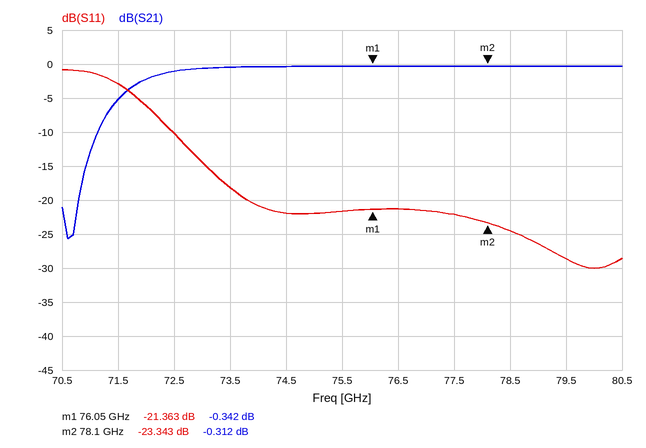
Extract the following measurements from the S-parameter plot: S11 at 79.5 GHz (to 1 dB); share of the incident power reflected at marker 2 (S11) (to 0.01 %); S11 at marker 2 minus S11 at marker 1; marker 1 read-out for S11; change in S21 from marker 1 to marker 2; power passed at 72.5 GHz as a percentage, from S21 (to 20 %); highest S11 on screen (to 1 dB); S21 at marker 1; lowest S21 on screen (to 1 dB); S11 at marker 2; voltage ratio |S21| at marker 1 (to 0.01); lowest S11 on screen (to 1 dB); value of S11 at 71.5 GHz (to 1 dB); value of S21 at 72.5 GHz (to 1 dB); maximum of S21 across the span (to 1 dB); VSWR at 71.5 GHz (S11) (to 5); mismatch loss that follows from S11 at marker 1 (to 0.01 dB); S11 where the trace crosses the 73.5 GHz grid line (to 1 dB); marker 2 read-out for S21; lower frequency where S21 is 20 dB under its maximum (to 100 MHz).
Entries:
-29 dB
0.46 %
-1.980 dB
-21.363 dB
0.030 dB
80 %
-1 dB
-0.342 dB
-26 dB
-23.343 dB
0.96
-30 dB
-3 dB
-1 dB
0 dB
5
0.03 dB
-18 dB
-0.312 dB
70.8 GHz
